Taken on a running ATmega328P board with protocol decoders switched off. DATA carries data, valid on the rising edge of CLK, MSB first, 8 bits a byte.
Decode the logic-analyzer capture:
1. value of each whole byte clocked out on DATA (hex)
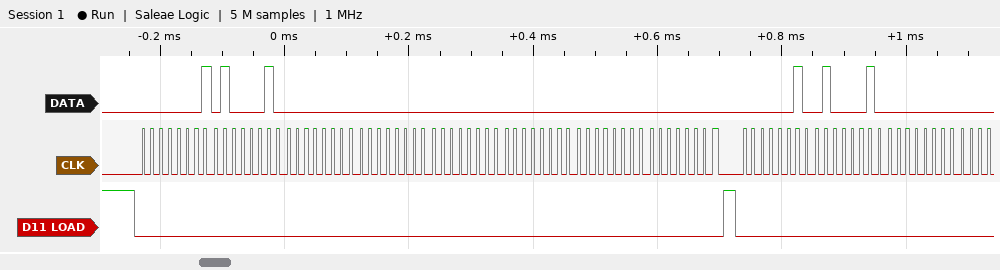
01 42 00 00 00 00 00 00 02 42 00
